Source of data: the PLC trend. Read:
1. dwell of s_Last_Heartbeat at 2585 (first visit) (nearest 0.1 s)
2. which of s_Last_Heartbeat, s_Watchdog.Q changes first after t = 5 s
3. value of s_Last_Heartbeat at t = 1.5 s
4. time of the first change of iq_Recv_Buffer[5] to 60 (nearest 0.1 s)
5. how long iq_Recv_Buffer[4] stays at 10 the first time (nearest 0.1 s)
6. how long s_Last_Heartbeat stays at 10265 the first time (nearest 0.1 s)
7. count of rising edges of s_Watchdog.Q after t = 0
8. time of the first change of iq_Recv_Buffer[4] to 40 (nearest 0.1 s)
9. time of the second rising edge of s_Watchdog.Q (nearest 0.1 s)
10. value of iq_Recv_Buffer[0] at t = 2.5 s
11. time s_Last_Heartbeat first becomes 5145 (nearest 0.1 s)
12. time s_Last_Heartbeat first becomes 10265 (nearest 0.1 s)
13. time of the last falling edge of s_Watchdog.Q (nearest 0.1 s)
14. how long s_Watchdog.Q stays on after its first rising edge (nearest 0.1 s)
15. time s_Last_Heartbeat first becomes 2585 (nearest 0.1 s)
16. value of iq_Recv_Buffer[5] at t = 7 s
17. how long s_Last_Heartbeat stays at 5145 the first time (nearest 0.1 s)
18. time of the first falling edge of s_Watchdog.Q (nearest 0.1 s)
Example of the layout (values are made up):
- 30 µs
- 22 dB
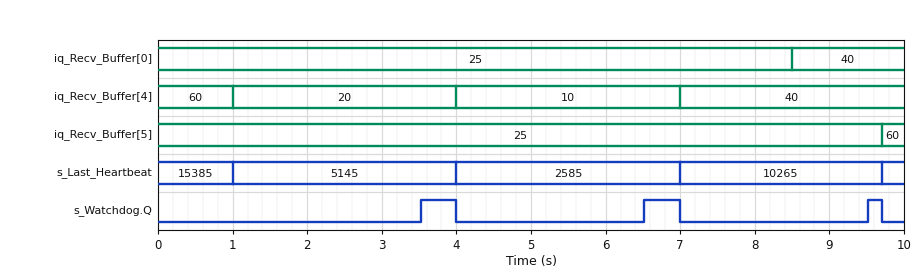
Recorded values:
- 3.0 s
- s_Watchdog.Q
- 5145
- 9.7 s
- 3.0 s
- 2.7 s
- 3
- 7.0 s
- 6.5 s
- 25
- 1.0 s
- 7.0 s
- 9.7 s
- 0.5 s
- 4.0 s
- 25
- 3.0 s
- 4.0 s
